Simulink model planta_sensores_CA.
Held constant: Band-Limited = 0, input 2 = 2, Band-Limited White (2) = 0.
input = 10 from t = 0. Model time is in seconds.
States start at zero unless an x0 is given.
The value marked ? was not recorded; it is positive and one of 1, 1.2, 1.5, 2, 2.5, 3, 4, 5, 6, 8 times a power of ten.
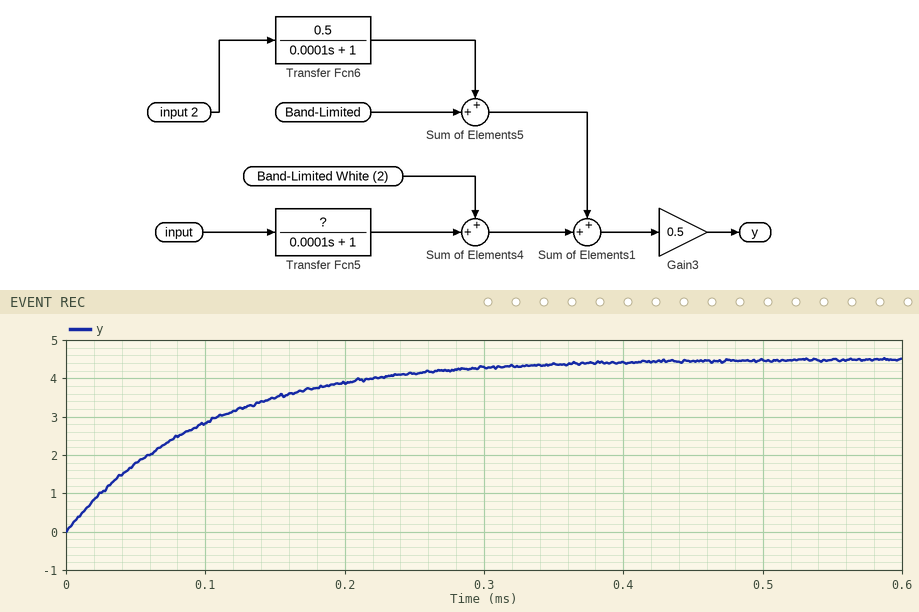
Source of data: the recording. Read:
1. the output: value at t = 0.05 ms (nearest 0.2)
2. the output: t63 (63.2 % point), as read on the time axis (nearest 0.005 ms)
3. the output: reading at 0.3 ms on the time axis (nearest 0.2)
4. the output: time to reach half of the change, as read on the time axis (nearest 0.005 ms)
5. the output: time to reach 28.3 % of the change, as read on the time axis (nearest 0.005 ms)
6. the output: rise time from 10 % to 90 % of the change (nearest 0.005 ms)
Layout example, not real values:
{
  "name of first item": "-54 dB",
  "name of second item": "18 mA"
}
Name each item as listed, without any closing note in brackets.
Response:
{
  "the output: value at t = 0.05 ms": "1.8",
  "the output: t63 (63.2 % point), as read on the time axis": "0.100 ms",
  "the output: reading at 0.3 ms on the time axis": "4.2",
  "the output: time to reach half of the change, as read on the time axis": "0.070 ms",
  "the output: time to reach 28.3 % of the change, as read on the time axis": "0.035 ms",
  "the output: rise time from 10 % to 90 % of the change": "0.220 ms"
}
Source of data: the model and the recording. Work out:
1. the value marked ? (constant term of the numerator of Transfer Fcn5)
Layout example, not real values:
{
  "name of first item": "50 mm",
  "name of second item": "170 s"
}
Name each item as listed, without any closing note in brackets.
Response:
{
  "the value marked ?": "0.8"
}
